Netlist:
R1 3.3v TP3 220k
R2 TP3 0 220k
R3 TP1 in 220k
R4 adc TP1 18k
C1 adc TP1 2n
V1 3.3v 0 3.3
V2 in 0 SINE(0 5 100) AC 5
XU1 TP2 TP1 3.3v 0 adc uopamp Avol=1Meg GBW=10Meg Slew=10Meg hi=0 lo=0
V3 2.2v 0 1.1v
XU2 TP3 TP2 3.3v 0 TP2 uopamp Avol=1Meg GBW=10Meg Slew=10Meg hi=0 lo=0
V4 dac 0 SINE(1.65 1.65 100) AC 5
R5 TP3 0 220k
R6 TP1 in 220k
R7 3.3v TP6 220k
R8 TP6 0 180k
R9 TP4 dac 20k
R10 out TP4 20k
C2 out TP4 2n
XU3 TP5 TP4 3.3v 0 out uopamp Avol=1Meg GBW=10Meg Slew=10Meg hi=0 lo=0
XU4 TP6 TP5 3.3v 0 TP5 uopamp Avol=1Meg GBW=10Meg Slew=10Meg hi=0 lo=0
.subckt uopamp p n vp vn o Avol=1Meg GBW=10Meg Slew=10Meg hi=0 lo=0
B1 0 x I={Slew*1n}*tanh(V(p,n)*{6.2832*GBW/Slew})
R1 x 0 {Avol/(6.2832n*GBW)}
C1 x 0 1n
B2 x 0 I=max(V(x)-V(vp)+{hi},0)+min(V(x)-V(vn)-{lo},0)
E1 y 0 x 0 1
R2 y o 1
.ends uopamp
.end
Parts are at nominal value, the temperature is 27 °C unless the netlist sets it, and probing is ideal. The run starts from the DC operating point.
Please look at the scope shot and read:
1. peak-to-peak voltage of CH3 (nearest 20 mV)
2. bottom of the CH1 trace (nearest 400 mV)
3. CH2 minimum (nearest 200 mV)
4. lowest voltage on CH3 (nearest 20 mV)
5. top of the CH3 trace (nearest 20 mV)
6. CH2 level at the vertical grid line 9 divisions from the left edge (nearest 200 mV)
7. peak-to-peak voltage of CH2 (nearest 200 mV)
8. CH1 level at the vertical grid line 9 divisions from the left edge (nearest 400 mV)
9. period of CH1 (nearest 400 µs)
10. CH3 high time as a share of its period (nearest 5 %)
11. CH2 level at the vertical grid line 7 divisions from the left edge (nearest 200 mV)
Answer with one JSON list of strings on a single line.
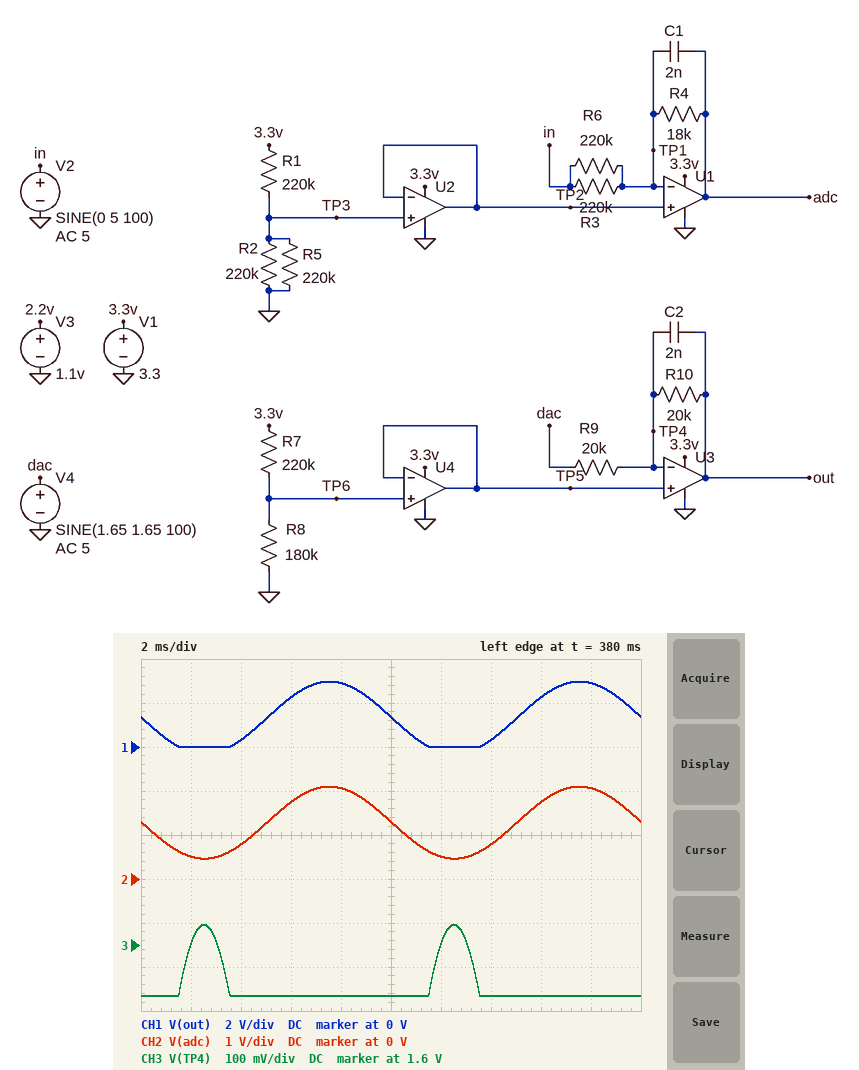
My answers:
["160 mV", "0 V", "400 mV", "1.48 V", "1.64 V", "2.0 V", "1.6 V", "2.8 V", "10.0 ms", "15 %", "800 mV"]
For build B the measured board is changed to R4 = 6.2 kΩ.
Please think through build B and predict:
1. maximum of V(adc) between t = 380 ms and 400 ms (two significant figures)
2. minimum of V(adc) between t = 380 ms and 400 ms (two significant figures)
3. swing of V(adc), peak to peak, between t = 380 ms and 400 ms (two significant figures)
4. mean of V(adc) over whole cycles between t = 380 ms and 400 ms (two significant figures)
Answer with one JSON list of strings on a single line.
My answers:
["1.4 V", "880 mV", "560 mV", "1.2 V"]
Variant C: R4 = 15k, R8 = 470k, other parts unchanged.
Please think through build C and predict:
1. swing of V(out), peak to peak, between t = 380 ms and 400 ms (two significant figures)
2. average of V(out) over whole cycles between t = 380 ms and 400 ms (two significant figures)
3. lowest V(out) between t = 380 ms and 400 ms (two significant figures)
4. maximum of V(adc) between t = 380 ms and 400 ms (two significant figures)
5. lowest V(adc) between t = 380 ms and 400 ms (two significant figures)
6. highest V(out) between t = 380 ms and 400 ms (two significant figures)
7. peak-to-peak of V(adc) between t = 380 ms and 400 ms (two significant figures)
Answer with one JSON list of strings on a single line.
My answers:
["2.1 V", "2.5 V", "1.2 V", "1.9 V", "570 mV", "3.3 V", "1.4 V"]
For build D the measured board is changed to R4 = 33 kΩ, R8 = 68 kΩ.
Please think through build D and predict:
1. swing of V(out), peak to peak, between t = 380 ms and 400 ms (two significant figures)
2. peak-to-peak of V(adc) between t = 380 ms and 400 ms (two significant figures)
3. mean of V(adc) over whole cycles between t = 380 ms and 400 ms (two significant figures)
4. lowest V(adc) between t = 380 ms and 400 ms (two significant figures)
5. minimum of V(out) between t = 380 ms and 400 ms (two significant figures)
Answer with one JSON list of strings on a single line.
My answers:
["1.6 V", "2.9 V", "1.4 V", "-3.1 mV", "-9.9 mV"]
